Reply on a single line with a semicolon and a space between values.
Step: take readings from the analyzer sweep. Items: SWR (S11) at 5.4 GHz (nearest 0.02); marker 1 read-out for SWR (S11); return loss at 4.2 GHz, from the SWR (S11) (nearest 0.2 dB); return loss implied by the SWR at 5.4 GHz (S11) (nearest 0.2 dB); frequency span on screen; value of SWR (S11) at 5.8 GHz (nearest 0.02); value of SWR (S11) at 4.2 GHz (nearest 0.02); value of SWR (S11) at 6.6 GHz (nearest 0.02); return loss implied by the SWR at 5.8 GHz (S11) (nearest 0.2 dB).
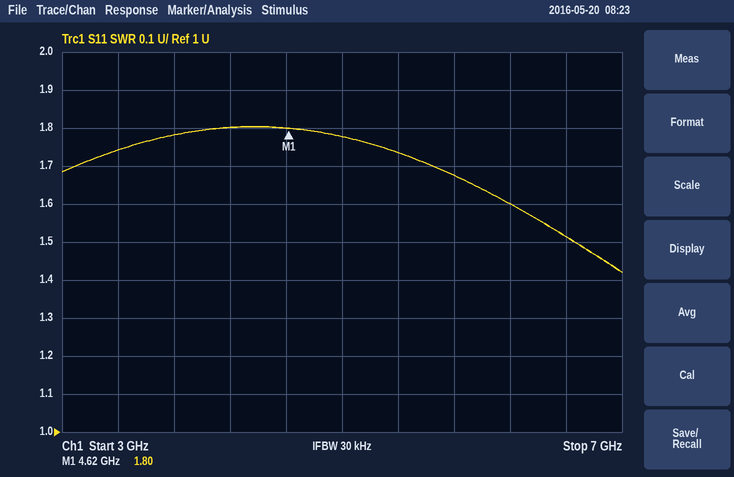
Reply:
1.74; 1.80; 10.8 dB; 11.4 dB; 4 GHz; 1.68; 1.80; 1.52; 12.0 dB
